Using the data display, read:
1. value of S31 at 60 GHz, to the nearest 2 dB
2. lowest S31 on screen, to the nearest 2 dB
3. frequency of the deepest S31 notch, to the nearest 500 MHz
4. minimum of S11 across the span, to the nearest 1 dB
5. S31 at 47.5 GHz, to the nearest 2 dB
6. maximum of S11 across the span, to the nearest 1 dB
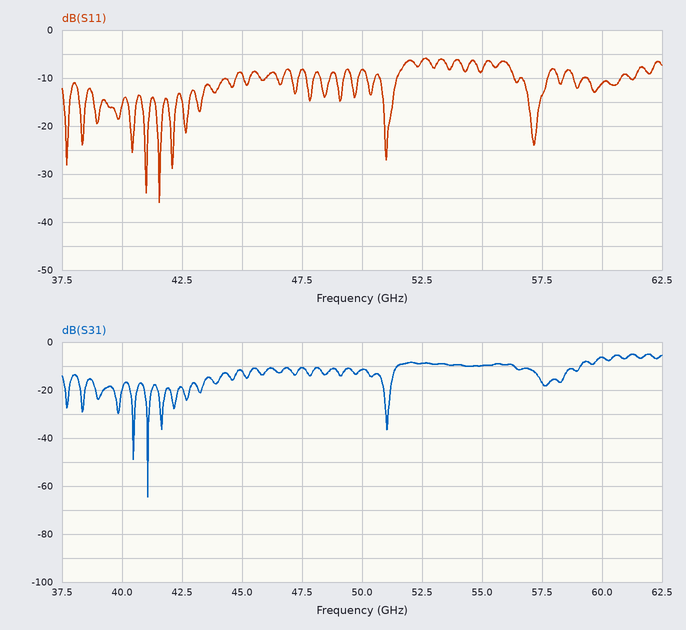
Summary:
-6 dB
-64 dB
41.0 GHz
-36 dB
-10 dB
-6 dB
